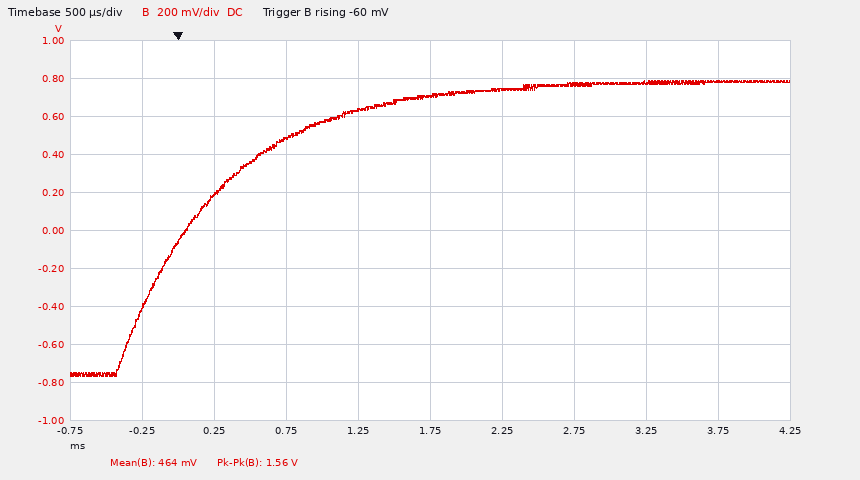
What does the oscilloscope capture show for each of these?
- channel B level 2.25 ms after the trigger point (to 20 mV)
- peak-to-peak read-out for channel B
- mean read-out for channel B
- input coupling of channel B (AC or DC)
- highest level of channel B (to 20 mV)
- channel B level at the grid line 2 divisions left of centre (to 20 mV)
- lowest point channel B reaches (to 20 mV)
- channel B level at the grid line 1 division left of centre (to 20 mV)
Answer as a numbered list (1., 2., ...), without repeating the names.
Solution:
1. 740 mV
2. 1.56 V
3. 464 mV
4. DC
5. 780 mV
6. 480 mV
7. -760 mV
8. 640 mV
